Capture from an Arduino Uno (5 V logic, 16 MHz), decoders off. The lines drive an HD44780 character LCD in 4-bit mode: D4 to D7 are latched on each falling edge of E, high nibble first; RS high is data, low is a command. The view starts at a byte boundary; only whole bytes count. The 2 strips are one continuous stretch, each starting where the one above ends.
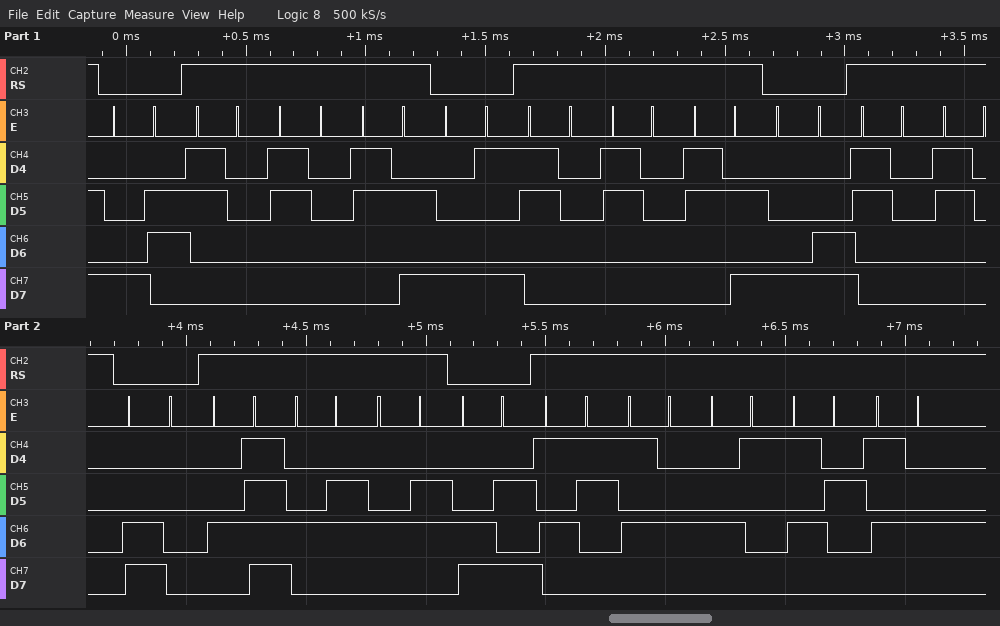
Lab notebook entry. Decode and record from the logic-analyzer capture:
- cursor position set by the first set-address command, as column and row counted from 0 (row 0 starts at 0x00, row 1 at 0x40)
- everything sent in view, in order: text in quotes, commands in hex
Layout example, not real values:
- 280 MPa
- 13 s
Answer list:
- column 6, row 0
- 0x86 "00:" 0x89 "00:" 0x8C "00" 0xC0 "OFF" 0xCA "START"
